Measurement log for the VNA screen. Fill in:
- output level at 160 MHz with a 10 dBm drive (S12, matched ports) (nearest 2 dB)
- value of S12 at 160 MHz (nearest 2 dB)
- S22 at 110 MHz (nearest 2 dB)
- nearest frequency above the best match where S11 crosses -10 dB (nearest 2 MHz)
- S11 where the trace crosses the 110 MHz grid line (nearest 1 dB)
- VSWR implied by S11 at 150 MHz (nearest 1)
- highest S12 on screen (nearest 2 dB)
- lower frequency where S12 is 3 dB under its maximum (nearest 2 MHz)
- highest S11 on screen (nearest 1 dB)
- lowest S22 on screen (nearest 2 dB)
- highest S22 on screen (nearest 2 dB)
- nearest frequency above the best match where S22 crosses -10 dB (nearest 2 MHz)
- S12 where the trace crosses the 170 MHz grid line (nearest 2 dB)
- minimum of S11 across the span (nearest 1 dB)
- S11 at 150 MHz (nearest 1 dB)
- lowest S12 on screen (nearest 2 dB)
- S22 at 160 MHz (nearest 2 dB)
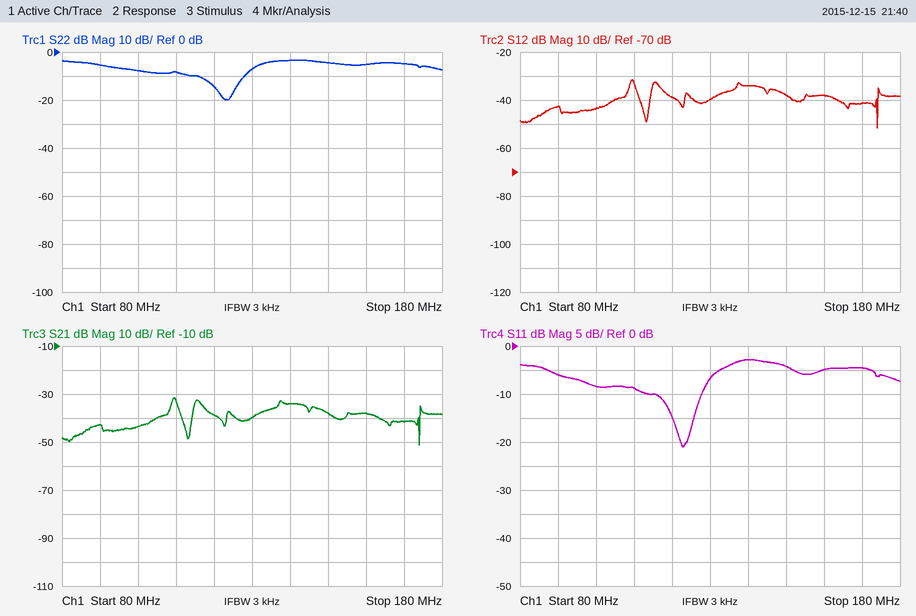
-28 dBm
-38 dB
-8 dB
128 MHz
-9 dB
4
-32 dB
108 MHz
-3 dB
-20 dB
-4 dB
128 MHz
-42 dB
-21 dB
-4 dB
-52 dB
-6 dB
